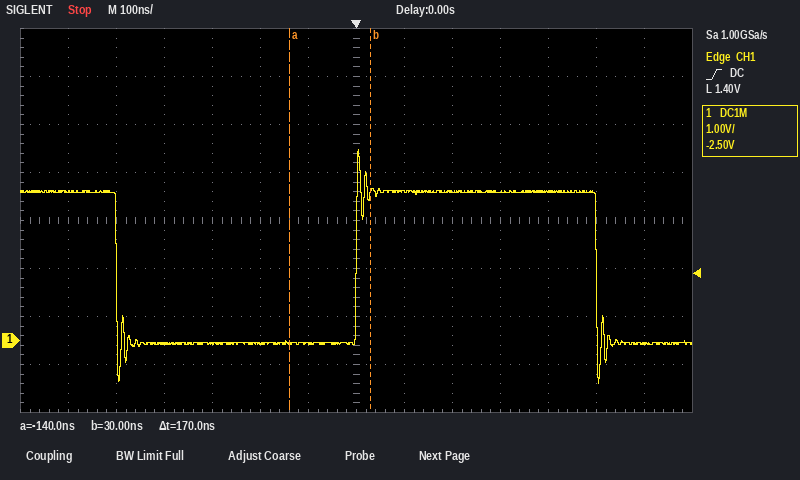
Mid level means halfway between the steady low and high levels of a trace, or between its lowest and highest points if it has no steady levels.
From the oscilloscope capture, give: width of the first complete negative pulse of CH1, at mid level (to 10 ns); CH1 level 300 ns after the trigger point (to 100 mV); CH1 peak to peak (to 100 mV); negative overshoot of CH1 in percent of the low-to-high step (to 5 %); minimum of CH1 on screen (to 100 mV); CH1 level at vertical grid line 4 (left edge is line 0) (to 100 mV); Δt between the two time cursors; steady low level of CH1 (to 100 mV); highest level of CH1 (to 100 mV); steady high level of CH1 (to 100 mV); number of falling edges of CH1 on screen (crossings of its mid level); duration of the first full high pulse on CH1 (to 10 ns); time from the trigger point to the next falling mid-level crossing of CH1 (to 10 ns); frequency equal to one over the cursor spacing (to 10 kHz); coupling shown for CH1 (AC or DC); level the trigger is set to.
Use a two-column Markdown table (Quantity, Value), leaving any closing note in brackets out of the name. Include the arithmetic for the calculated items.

| Quantity | Value |
|---|---|
| width of the first complete negative pulse of CH1, at mid level | 500 ns |
| CH1 level 300 ns after the trigger point | 3.1 V |
| CH1 peak to peak | 4.0 V − (-900 mV) = 4.9 V |
| negative overshoot of CH1 in percent of the low-to-high step | 25 % |
| minimum of CH1 on screen | -900 mV |
| CH1 level at vertical grid line 4 (left edge is line 0) | -100 mV |
| Δt between the two time cursors | 170 ns |
| steady low level of CH1 | -100 mV |
| highest level of CH1 | 4.0 V |
| steady high level of CH1 | 3.1 V |
| number of falling edges of CH1 on screen | 2 |
| duration of the first full high pulse on CH1 | 500 ns |
| time from the trigger point to the next falling mid-level crossing of CH1 | 500 ns |
| frequency equal to one over the cursor spacing | 1 / 170 ns ≈ 5.88 MHz |
| coupling shown for CH1 | DC |
| level the trigger is set to | 1.40 V |
